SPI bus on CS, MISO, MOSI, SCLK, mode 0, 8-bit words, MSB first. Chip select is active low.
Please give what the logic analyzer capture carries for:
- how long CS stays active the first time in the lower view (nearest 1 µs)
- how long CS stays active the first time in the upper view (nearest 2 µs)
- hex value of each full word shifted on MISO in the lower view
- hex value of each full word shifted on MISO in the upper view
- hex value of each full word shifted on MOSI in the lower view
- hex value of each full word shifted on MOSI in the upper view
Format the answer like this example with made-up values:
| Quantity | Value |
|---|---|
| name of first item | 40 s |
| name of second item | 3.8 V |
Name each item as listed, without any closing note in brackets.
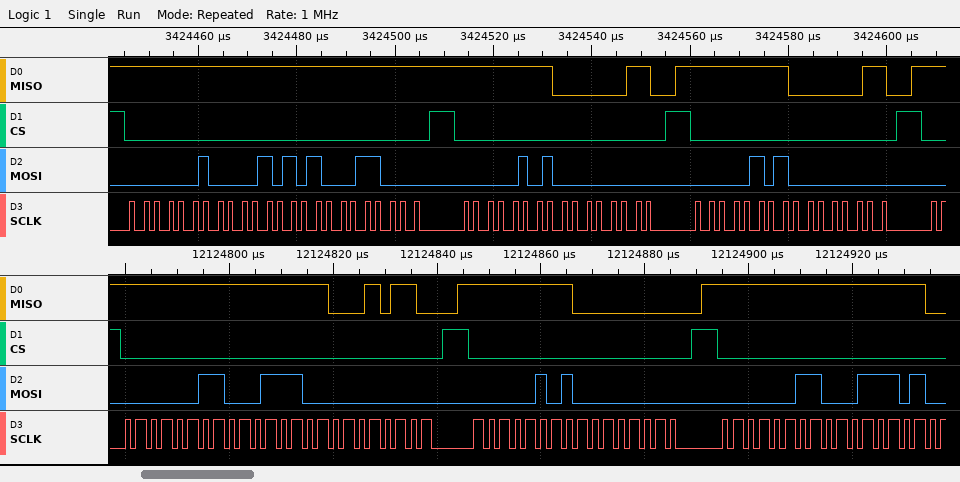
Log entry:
| Quantity | Value |
|---|---|
| how long CS stays active the first time in the lower view | 62 µs |
| how long CS stays active the first time in the upper view | 62 µs |
| hex value of each full word shifted on MISO in the lower view | FF, FF, 16, FF, 00, FF, FF |
| hex value of each full word shifted on MISO in the upper view | FF, FF, FF, FF, 03, FF, 03 |
| hex value of each full word shifted on MOSI in the lower view | 03, 1C, 00, 05, 00, 03, 1D |
| hex value of each full word shifted on MOSI in the upper view | 02, 15, 18, 05, 00, 05, 00 |
